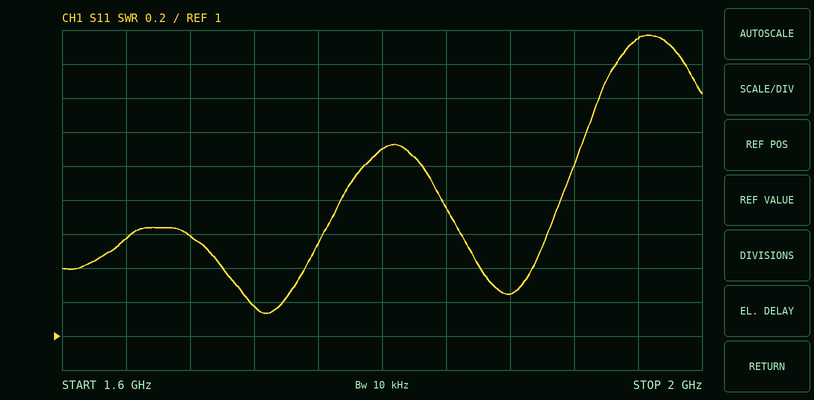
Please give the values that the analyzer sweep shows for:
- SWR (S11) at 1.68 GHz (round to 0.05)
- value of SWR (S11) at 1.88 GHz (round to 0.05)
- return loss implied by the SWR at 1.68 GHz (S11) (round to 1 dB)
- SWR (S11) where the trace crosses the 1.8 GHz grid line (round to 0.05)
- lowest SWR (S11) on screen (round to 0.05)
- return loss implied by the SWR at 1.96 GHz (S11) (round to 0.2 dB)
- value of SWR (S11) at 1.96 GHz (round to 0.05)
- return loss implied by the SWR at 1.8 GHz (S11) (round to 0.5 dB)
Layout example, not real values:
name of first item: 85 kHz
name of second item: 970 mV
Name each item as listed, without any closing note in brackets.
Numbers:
SWR (S11) at 1.68 GHz: 1.60
value of SWR (S11) at 1.88 GHz: 1.25
return loss implied by the SWR at 1.68 GHz (S11): 13 dB
SWR (S11) where the trace crosses the 1.8 GHz grid line: 2.10
lowest SWR (S11) on screen: 1.15
return loss implied by the SWR at 1.96 GHz (S11): 6.6 dB
value of SWR (S11) at 1.96 GHz: 2.75
return loss implied by the SWR at 1.8 GHz (S11): 9.0 dB
